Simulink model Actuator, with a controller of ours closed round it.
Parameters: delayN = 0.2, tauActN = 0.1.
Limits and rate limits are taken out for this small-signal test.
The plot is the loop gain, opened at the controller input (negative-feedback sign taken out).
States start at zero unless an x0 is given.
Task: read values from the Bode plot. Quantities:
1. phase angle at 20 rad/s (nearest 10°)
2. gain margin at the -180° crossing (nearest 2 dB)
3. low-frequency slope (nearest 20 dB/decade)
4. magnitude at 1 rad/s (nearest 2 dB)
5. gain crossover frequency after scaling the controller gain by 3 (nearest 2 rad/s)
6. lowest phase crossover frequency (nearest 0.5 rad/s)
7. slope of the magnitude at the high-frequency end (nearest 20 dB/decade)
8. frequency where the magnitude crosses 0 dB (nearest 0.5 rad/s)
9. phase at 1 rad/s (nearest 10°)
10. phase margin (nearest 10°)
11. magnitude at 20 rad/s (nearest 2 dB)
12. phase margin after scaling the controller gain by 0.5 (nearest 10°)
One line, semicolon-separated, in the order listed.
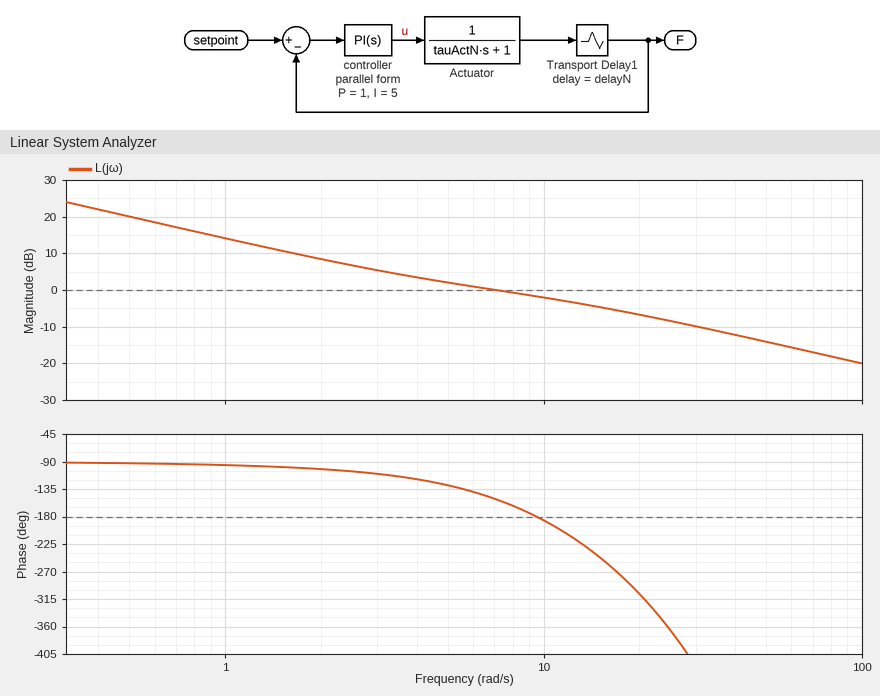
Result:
-310°; 2 dB; -20 dB/decade; 14 dB; 28 rad/s; 9.5 rad/s; -20 dB/decade; 7.0 rad/s; -100°; 30°; -6 dB; 70°
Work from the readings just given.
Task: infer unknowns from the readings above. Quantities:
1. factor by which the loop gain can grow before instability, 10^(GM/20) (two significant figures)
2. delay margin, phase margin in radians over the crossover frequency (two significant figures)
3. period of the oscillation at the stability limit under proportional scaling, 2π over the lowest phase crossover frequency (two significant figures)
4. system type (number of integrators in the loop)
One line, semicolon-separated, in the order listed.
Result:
1.3; 0.075 s; 0.66 s; 1
